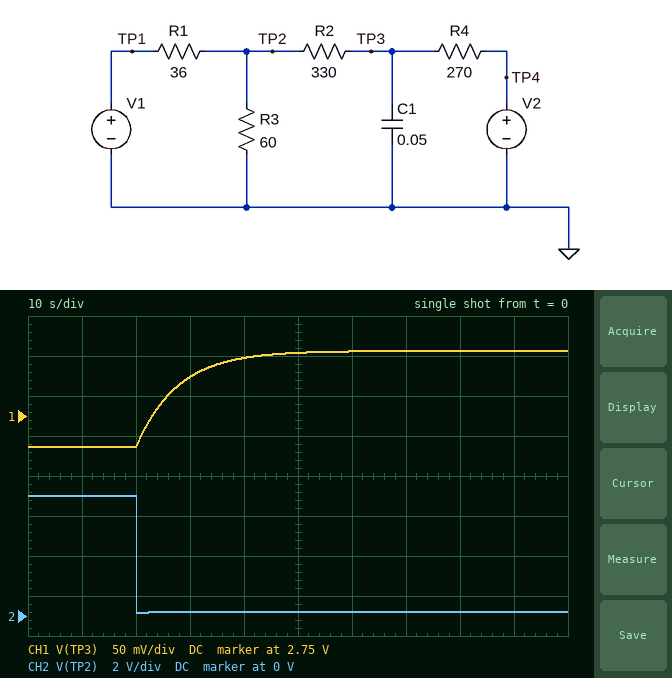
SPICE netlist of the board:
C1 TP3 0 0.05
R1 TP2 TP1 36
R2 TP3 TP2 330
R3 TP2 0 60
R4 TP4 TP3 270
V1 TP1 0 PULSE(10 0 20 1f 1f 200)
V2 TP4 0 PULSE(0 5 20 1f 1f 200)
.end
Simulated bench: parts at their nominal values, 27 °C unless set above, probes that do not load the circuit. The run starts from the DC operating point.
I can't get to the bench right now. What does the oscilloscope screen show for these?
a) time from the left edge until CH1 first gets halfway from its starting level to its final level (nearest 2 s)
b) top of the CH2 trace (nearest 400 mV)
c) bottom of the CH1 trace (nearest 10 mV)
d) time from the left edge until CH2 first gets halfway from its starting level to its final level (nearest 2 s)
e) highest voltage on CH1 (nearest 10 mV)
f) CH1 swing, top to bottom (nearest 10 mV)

26 s
6.0 V
2.71 V
20 s
2.83 V
120 mV
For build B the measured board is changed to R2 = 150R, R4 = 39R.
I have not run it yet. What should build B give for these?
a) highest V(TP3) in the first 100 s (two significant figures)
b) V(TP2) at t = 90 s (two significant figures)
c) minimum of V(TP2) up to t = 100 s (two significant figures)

4.1 V
530 mV
150 mV
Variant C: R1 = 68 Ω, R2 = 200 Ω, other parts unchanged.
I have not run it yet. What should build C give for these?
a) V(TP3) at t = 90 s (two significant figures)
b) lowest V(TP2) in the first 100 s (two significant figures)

2.3 V
320 mV
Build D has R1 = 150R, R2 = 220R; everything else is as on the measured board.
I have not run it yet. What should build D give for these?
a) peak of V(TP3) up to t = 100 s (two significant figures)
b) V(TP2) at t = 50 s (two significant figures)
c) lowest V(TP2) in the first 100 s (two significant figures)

2.5 V
400 mV
240 mV
